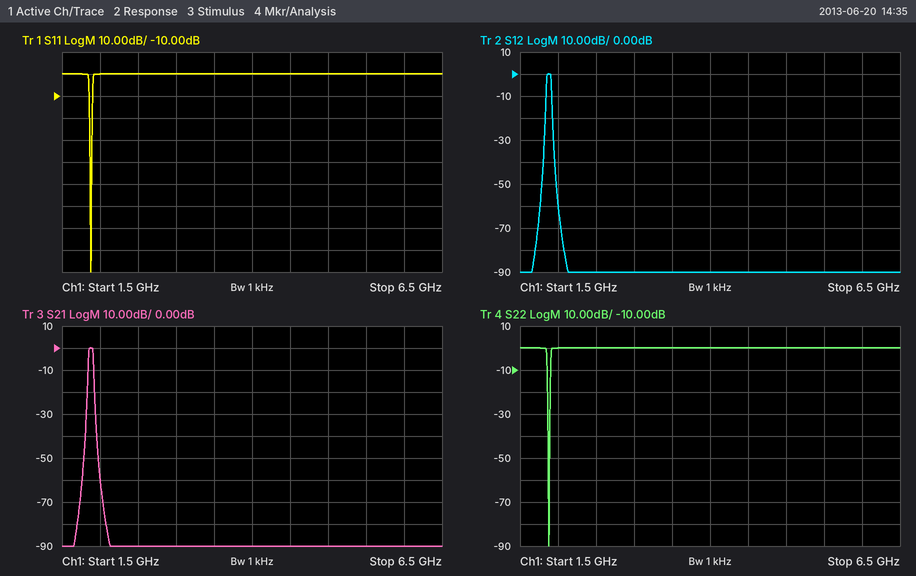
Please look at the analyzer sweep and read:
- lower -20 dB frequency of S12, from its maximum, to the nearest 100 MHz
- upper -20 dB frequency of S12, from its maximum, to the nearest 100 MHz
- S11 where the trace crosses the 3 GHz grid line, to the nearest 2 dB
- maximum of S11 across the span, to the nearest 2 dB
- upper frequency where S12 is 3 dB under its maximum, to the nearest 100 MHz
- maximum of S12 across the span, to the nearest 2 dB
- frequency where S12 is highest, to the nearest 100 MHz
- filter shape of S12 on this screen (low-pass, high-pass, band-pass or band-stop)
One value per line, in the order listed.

1.8 GHz
1.9 GHz
0 dB
0 dB
1.9 GHz
0 dB
1.9 GHz
band-pass
